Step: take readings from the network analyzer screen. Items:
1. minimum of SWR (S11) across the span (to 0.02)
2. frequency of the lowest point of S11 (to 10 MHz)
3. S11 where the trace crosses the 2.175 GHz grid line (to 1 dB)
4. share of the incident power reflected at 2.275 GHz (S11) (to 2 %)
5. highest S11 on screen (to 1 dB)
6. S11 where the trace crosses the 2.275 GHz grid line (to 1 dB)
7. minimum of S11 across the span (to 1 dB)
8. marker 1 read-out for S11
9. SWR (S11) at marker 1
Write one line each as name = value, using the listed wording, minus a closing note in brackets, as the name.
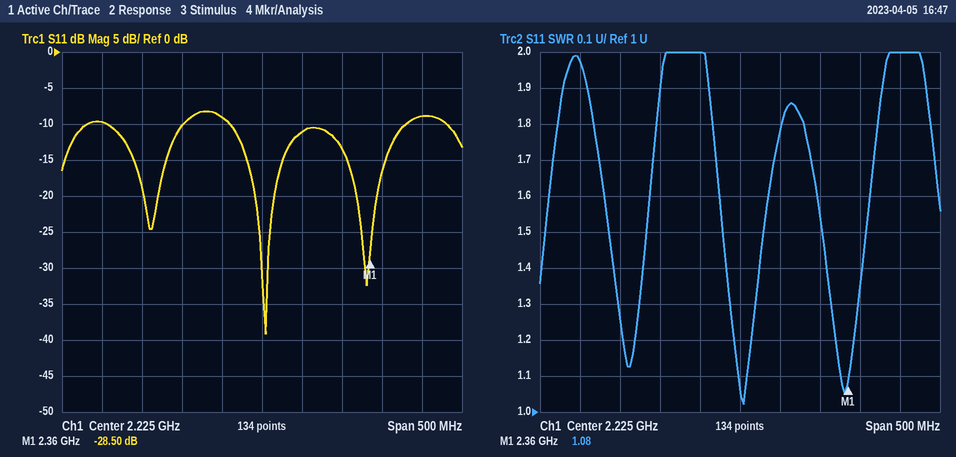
minimum of SWR (S11) across the span = 1.02
frequency of the lowest point of S11 = 2.23 GHz
S11 where the trace crosses the 2.175 GHz grid line = -9 dB
share of the incident power reflected at 2.275 GHz (S11) = 8 %
highest S11 on screen = -8 dB
S11 where the trace crosses the 2.275 GHz grid line = -11 dB
minimum of S11 across the span = -39 dB
marker 1 read-out for S11 = -28.50 dB
SWR (S11) at marker 1 = 1.08
